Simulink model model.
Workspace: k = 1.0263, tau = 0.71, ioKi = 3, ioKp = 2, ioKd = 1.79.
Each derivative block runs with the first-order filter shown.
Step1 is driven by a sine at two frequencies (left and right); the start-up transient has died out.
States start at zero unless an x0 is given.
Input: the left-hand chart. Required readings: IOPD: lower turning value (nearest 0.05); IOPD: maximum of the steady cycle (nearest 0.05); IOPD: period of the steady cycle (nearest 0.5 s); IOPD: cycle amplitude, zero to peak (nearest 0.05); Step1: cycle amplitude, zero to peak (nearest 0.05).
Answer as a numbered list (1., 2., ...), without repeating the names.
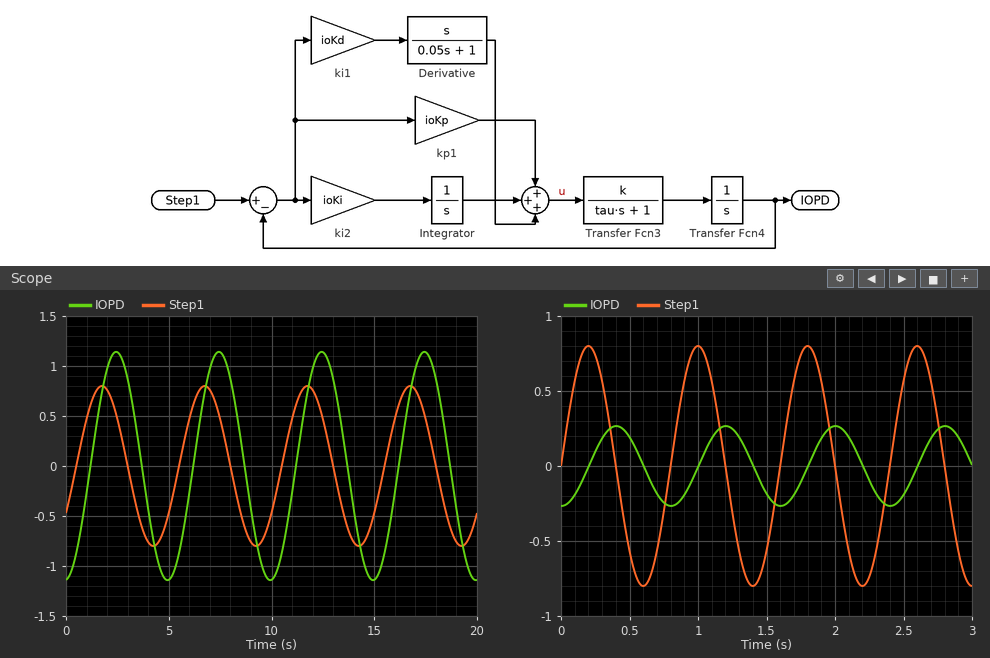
1. -1.15
2. 1.15
3. 5.0 s
4. 1.15
5. 0.80
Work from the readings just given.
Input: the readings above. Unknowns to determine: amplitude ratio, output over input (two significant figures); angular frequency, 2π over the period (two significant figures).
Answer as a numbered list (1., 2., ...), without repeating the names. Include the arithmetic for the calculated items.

1. 1.15 / 0.8 = 1.4
2. 2π / 5 = 1.3 rad/s
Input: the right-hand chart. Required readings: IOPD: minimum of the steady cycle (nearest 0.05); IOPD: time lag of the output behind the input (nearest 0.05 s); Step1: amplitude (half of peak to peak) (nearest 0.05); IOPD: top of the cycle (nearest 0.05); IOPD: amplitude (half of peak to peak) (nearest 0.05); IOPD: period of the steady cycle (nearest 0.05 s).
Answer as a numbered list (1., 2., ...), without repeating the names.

1. -0.25
2. 0.20 s
3. 0.80
4. 0.25
5. 0.25
6. 0.80 s
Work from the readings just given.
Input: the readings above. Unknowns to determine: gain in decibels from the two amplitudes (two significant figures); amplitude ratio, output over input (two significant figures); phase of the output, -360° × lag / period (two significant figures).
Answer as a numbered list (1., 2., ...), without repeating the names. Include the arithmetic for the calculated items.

1. 20 log10(0.25 / 0.8) = -10 dB
2. 0.25 / 0.8 = 0.31
3. -360 × 0.2 / 0.8 = -90°
